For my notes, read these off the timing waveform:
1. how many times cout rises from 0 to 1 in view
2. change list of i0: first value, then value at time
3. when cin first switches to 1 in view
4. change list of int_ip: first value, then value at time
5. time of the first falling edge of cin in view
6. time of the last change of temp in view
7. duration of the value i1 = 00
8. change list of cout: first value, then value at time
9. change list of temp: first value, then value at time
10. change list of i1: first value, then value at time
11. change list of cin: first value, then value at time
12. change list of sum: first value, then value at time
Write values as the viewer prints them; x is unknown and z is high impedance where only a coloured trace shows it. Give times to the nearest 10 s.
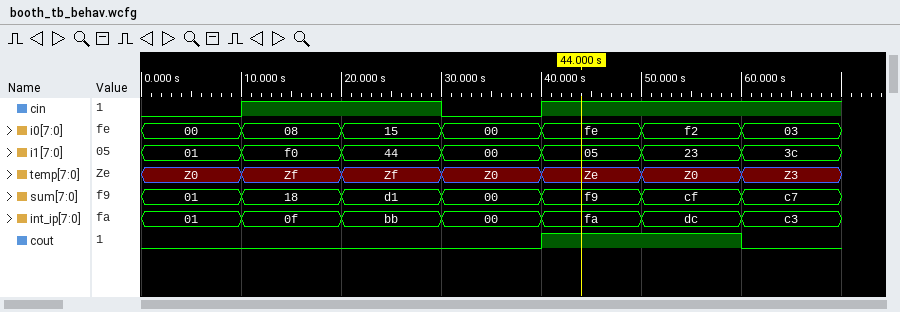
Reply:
1
00, 08 at 10 s, 15 at 20 s, 00 at 30 s, fe at 40 s, f2 at 50 s, 03 at 60 s
10 s
01, 0f at 10 s, bb at 20 s, 00 at 30 s, fa at 40 s, dc at 50 s, c3 at 60 s
30 s
60 s
10 s
0, 1 at 40 s, 0 at 60 s
Z0, Zf at 10 s, Zf at 20 s, Z0 at 30 s, Ze at 40 s, Z0 at 50 s, Z3 at 60 s
01, f0 at 10 s, 44 at 20 s, 00 at 30 s, 05 at 40 s, 23 at 50 s, 3c at 60 s
0, 1 at 10 s, 0 at 30 s, 1 at 40 s
01, 18 at 10 s, d1 at 20 s, 00 at 30 s, f9 at 40 s, cf at 50 s, c7 at 60 s
